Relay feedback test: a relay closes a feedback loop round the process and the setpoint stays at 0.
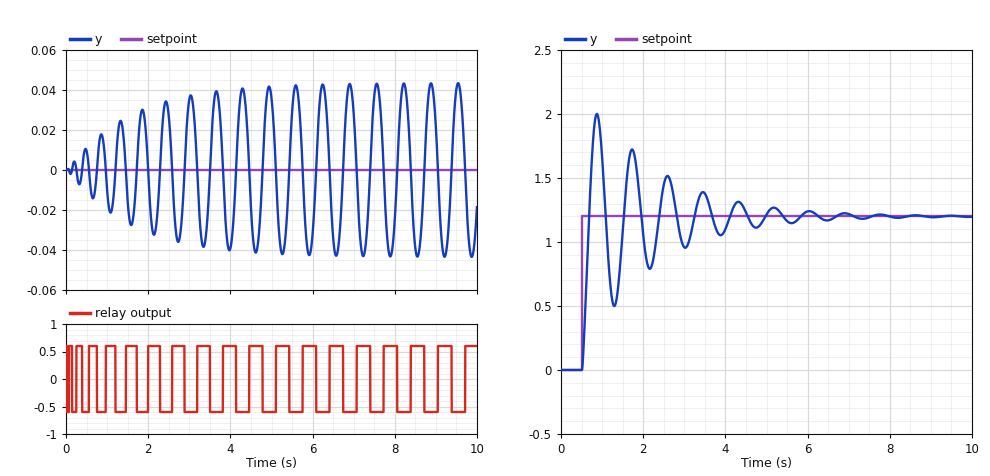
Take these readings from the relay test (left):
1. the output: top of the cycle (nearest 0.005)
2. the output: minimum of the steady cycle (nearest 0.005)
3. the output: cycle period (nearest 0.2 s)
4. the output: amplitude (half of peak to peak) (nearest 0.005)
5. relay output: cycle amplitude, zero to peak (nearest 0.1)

0.045
-0.045
0.6 s
0.045
0.6
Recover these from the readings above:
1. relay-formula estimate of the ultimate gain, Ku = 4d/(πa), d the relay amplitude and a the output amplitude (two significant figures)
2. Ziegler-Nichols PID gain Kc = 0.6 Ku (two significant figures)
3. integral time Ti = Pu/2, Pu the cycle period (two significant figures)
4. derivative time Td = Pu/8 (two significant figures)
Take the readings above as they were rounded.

17
10
0.30 s
0.075 s
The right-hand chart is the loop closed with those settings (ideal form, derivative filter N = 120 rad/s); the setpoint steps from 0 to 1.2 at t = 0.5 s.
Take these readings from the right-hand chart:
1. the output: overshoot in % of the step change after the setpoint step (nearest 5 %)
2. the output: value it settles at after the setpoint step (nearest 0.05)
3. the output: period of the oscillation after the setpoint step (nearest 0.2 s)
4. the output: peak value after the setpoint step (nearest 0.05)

65 %
1.20
0.8 s
2.00
